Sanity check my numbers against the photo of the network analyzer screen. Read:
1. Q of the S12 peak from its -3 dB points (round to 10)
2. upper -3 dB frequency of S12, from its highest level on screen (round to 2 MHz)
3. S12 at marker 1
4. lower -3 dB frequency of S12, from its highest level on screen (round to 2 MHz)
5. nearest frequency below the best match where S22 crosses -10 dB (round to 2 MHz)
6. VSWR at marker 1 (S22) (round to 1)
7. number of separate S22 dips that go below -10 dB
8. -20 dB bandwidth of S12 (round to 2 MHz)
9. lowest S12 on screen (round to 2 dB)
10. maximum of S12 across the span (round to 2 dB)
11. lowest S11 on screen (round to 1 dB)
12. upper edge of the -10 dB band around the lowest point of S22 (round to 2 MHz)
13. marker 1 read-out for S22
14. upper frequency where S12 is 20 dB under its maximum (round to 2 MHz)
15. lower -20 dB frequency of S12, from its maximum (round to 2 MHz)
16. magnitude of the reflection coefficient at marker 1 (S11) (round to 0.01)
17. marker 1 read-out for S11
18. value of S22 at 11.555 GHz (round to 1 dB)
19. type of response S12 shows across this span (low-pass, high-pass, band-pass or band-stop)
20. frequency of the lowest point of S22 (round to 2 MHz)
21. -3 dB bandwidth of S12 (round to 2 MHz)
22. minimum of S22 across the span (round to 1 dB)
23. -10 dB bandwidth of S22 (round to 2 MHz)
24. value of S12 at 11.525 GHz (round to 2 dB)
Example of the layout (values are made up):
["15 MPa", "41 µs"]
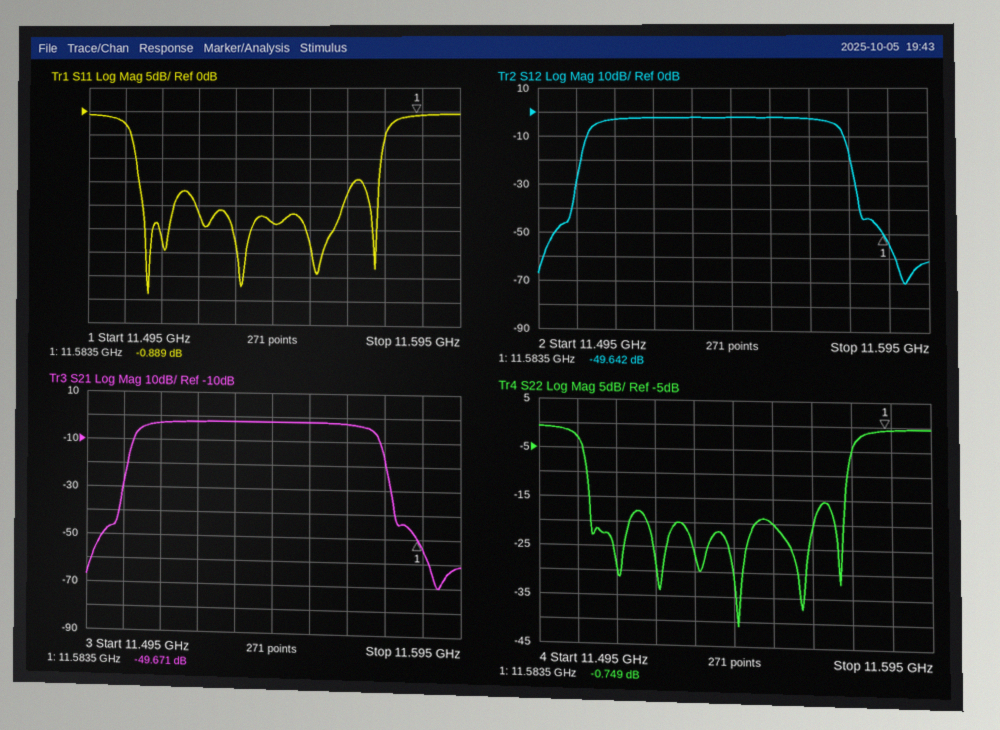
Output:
["190", "11.572 GHz", "-49.642 dB", "11.510 GHz", "11.508 GHz", "23", "6", "70 MHz", "-70 dB", "-2 dB", "-39 dB", "11.574 GHz", "-0.749 dB", "11.576 GHz", "11.506 GHz", "0.90", "-0.889 dB", "-20 dB", "band-pass", "11.546 GHz", "62 MHz", "-41 dB", "66 MHz", "-2 dB"]
